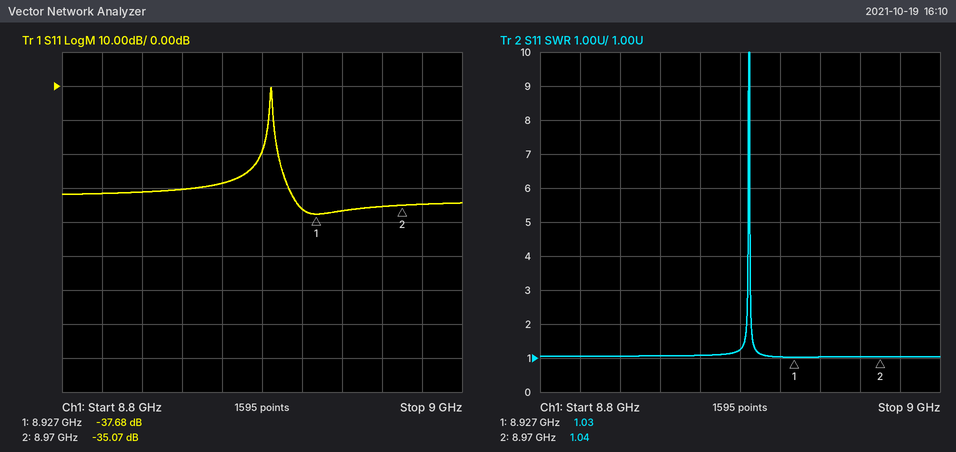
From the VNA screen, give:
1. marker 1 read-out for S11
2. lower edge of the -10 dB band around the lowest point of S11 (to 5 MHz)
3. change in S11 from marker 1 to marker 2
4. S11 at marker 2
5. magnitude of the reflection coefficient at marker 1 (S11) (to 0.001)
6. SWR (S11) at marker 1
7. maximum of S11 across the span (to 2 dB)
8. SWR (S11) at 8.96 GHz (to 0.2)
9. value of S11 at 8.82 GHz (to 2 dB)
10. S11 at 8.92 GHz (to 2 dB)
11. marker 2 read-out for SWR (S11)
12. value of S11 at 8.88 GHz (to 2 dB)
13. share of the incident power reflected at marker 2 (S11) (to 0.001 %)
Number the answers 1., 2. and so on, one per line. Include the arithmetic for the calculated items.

1. -37.68 dB
2. 8.905 GHz
3. -35.07 − (-37.68) = 2.61 dB
4. -35.07 dB
5. 10^(-37.68/20) ≈ 0.013
6. 1.03
7. 0 dB
8. 1.0
9. -32 dB
10. -36 dB
11. 1.04
12. -28 dB
13. 10^(-35.07/10) ≈ 0.031 %
